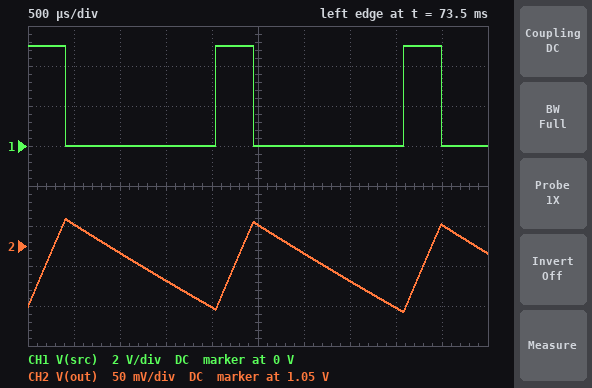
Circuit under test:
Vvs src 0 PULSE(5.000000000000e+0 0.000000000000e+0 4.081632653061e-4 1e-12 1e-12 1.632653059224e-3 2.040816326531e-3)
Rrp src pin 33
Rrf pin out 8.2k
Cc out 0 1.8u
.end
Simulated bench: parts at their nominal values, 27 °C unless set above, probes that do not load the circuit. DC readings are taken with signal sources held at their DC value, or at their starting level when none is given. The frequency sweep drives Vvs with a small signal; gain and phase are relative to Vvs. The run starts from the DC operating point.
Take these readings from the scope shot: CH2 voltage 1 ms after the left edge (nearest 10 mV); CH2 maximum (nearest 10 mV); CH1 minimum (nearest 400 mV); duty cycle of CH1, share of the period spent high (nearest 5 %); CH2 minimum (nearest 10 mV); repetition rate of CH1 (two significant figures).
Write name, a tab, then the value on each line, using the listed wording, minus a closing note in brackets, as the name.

CH2 voltage 1 ms after the left edge	1.04 V
CH2 maximum	1.08 V
CH1 minimum	0 V
duty cycle of CH1, share of the period spent high	20 %
CH2 minimum	970 mV
repetition rate of CH1	490 Hz
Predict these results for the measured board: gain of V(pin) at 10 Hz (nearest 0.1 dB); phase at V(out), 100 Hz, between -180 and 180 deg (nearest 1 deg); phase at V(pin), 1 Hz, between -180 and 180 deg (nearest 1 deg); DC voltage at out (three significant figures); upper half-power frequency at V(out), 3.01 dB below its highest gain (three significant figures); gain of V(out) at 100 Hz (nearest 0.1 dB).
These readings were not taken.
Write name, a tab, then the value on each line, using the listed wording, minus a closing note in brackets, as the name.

gain of V(pin) at 10 Hz	0 dB
phase at V(out), 100 Hz, between -180 and 180 deg	-84 deg
phase at V(pin), 1 Hz, between -180 and 180 deg	0 deg
DC voltage at out	5.00 V
upper half-power frequency at V(out), 3.01 dB below its highest gain	10.7 Hz
gain of V(out) at 100 Hz	-19.4 dB
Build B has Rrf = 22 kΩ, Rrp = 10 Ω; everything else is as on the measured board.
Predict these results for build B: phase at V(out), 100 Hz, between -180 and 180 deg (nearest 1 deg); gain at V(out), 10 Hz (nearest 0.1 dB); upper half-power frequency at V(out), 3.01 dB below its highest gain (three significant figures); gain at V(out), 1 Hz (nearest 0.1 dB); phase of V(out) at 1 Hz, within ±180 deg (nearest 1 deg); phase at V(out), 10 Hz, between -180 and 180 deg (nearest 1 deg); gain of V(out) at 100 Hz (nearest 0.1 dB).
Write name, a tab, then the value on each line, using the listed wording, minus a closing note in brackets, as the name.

phase at V(out), 100 Hz, between -180 and 180 deg	-88 deg
gain at V(out), 10 Hz	-8.6 dB
upper half-power frequency at V(out), 3.01 dB below its highest gain	4.02 Hz
gain at V(out), 1 Hz	-0.3 dB
phase of V(out) at 1 Hz, within ±180 deg	-14 deg
phase at V(out), 10 Hz, between -180 and 180 deg	-68 deg
gain of V(out) at 100 Hz	-27.9 dB
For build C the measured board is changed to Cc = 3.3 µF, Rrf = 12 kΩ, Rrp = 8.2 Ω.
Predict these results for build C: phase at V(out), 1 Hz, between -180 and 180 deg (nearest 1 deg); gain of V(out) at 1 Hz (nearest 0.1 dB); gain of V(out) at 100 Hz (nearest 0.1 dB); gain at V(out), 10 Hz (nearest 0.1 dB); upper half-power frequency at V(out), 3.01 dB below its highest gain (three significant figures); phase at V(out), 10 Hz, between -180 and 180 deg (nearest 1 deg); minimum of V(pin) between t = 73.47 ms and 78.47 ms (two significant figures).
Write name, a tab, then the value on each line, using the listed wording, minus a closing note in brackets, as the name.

phase at V(out), 1 Hz, between -180 and 180 deg	-14 deg
gain of V(out) at 1 Hz	-0.3 dB
gain of V(out) at 100 Hz	-27.9 dB
gain at V(out), 10 Hz	-8.6 dB
upper half-power frequency at V(out), 3.01 dB below its highest gain	4.02 Hz
phase at V(out), 10 Hz, between -180 and 180 deg	-68 deg
minimum of V(pin) between t = 73.47 ms and 78.47 ms	1.1 mV
